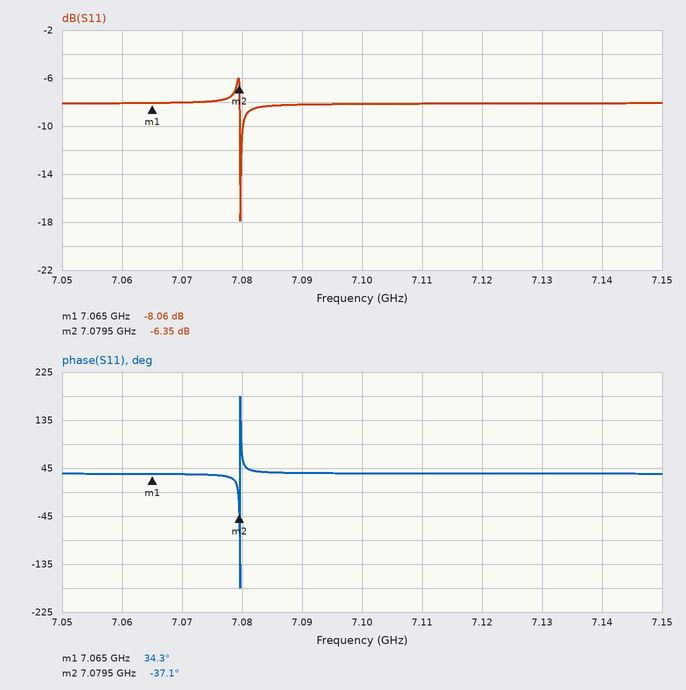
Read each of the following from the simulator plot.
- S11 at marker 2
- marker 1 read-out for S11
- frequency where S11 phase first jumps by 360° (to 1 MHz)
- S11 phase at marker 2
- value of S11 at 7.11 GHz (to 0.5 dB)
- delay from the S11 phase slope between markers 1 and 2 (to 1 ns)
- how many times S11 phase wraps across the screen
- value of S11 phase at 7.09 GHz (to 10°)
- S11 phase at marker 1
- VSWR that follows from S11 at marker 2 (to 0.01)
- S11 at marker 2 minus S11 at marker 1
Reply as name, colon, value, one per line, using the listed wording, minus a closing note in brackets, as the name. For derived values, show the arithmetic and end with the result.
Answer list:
S11 at marker 2: -6.35 dB
marker 1 read-out for S11: -8.06 dB
frequency where S11 phase first jumps by 360°: 7.080 GHz
S11 phase at marker 2: -37.1°
value of S11 at 7.11 GHz: -8.0 dB
delay from the S11 phase slope between markers 1 and 2: −(-37.1° − (34.3°))/(360° × 14.5 MHz) ≈ 14 ns
how many times S11 phase wraps across the screen: 1
value of S11 phase at 7.09 GHz: 40°
S11 phase at marker 1: 34.3°
VSWR that follows from S11 at marker 2: (1 + 0.4814)/(1 − 0.4814) ≈ 2.86
S11 at marker 2 minus S11 at marker 1: -6.35 − (-8.06) = 1.71 dB
